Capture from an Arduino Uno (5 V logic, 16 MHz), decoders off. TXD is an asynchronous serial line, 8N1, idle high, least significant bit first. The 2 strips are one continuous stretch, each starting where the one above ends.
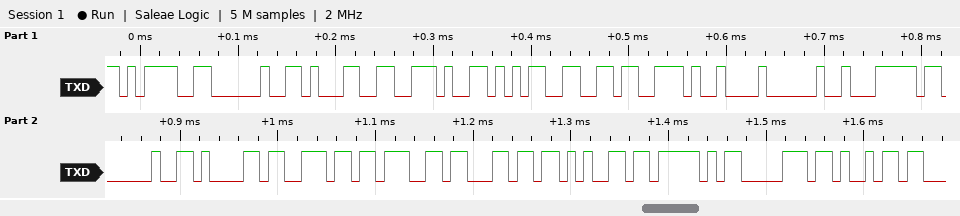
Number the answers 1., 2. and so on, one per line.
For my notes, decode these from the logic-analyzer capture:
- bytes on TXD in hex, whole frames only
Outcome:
1. 3D 20 31 2E 35 36 09 20 7C 20 61 6E 67 6C 65 5F 70 69
